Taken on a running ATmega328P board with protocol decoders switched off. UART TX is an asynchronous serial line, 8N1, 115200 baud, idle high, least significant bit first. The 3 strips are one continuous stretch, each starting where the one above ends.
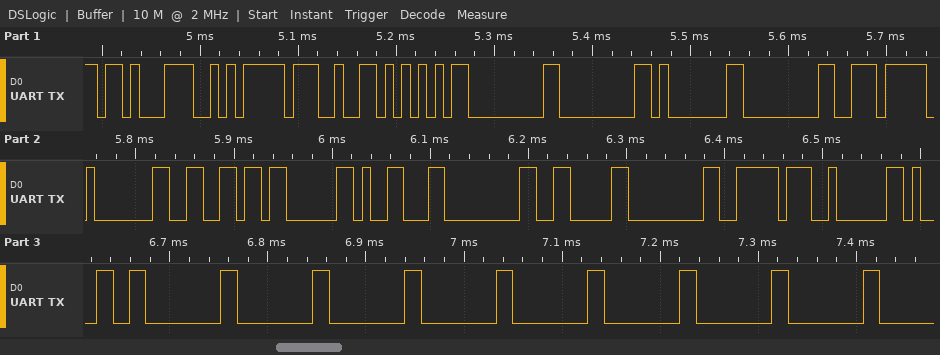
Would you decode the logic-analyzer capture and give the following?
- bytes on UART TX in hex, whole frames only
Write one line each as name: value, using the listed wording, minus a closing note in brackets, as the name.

bytes on UART TX in hex, whole frames only: 8B EA 27 55 00 00 01 00 EE 01 66 03 19 00 06 00 BE 02 31 00 00 00 00 00 00 00 00
